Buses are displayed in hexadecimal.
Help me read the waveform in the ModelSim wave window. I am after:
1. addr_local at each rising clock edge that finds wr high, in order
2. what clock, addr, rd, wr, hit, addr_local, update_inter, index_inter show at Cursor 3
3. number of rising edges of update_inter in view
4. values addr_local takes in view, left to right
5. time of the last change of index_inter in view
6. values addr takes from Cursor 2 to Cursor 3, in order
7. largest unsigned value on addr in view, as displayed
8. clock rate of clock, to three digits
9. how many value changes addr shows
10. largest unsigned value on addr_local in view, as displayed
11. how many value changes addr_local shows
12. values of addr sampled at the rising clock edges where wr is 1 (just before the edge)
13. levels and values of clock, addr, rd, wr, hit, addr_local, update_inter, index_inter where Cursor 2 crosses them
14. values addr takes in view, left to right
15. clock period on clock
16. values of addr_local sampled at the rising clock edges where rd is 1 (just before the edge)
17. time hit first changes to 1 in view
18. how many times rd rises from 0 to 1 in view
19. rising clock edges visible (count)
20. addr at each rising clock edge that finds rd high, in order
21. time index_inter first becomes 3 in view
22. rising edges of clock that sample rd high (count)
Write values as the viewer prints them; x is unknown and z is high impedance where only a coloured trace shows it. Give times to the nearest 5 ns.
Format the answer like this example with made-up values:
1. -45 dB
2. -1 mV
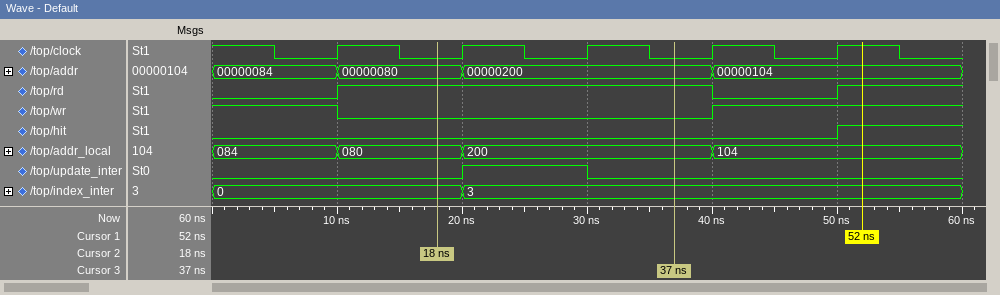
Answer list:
1. 084, 104
2. clock=0, addr=00000200, rd=1, wr=0, hit=0, addr_local=200, update_inter=0, index_inter=3
3. 1
4. 084, 080, 200, 104
5. 20 ns
6. 00000080, 00000200
7. 00000200
8. 100 MHz
9. 3
10. 200
11. 3
12. 00000084, 00000104
13. clock=0, addr=00000080, rd=1, wr=0, hit=0, addr_local=080, update_inter=0, index_inter=0
14. 00000084, 00000080, 00000200, 00000104
15. 10 ns
16. 080, 200, 200
17. 50 ns
18. 2
19. 5
20. 00000080, 00000200, 00000200
21. 20 ns
22. 3
